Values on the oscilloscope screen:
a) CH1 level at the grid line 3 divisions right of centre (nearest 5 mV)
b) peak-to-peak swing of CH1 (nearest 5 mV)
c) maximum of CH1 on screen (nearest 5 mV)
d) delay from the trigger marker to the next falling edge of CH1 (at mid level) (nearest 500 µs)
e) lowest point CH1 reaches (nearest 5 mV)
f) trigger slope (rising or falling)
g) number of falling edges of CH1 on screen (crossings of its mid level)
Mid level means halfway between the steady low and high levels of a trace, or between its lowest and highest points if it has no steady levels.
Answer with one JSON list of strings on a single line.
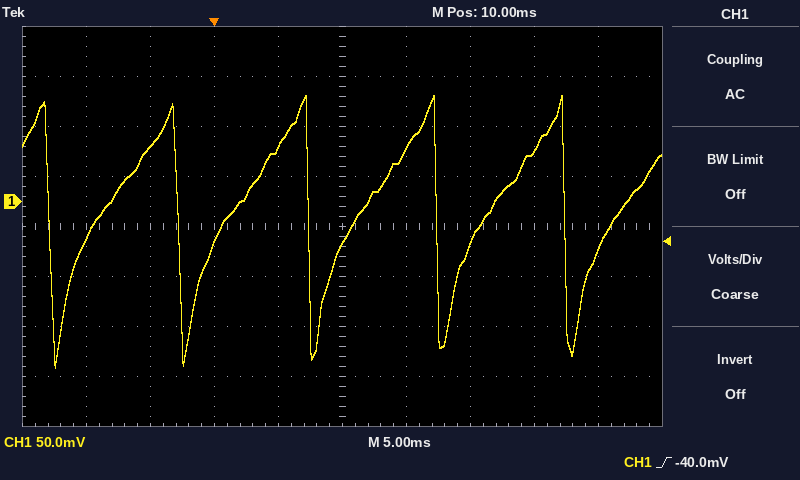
["50 mV", "270 mV", "105 mV", "7.5 ms", "-165 mV", "rising", "5"]
